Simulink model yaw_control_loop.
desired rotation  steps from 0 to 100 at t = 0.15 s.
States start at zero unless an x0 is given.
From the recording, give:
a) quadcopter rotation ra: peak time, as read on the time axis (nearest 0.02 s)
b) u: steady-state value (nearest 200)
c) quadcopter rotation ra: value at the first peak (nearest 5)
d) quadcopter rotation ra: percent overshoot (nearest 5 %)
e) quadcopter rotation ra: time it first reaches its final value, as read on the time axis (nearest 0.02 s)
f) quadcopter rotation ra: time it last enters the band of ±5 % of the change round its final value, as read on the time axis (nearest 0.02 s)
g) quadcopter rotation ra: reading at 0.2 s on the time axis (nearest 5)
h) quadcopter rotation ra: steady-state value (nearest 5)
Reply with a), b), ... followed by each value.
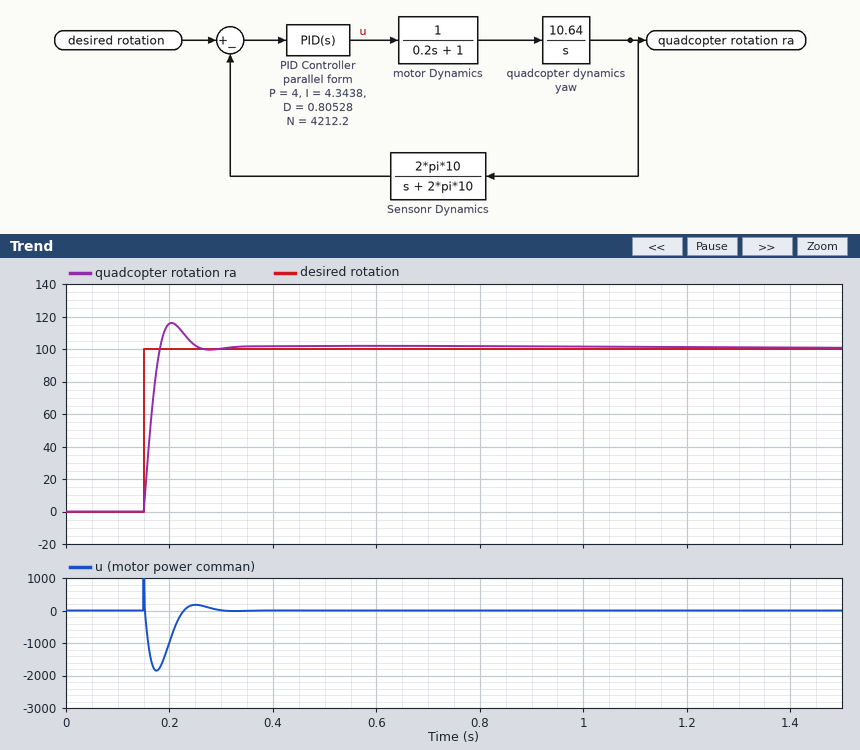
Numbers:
a) 0.20 s
b) 0
c) 115
d) 15 %
e) 0.18 s
f) 0.24 s
g) 115
h) 100
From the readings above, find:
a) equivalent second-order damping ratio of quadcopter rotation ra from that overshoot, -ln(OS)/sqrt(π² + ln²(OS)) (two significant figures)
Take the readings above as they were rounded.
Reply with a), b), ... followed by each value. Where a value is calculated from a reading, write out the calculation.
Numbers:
a) ln(0.15) = -1.897; 1.897 / sqrt(9.870 + 3.599) = 0.52
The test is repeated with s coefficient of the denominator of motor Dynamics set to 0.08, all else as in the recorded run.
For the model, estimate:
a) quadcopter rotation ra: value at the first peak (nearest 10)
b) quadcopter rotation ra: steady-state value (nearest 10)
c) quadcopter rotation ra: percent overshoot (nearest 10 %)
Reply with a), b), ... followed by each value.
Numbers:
a) 150
b) 100
c) 50 %
